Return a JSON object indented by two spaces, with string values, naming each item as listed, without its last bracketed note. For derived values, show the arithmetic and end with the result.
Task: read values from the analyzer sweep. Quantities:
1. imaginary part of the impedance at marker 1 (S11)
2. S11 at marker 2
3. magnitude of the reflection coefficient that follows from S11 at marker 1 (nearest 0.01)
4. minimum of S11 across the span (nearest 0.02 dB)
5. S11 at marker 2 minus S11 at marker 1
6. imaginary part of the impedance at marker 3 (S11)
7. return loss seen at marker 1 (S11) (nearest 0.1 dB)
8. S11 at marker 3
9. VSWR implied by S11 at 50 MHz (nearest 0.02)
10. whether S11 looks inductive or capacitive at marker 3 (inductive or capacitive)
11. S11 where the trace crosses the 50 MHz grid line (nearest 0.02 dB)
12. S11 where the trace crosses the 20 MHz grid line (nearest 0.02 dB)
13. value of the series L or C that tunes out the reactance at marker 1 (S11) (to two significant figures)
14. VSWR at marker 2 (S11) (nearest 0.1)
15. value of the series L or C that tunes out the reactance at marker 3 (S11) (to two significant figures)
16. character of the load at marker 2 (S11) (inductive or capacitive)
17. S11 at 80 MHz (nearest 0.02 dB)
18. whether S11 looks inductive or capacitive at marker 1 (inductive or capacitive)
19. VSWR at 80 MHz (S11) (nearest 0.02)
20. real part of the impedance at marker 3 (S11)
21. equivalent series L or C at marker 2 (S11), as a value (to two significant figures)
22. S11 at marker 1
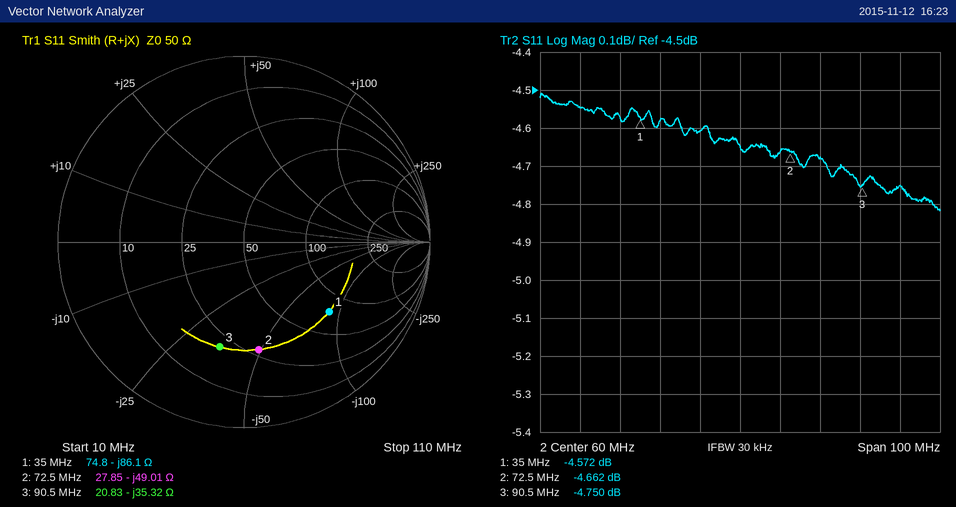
{
  "imaginary part of the impedance at marker 1": "-86.1 Ω",
  "S11 at marker 2": "-4.662 dB",
  "magnitude of the reflection coefficient that follows from S11 at marker 1": "10^(-4.572/20) ≈ 0.59",
  "minimum of S11 across the span": "-4.82 dB",
  "S11 at marker 2 minus S11 at marker 1": "-4.662 − (-4.572) = -0.090 dB",
  "imaginary part of the impedance at marker 3": "-35.32 Ω",
  "return loss seen at marker 1 (S11)": "4.6 dB",
  "S11 at marker 3": "-4.750 dB",
  "VSWR implied by S11 at 50 MHz": "|Γ| = 10^(-4.6/20) = 0.5888; VSWR = (1 + 0.5888)/(1 − 0.5888) ≈ 3.86",
  "whether S11 looks inductive or capacitive at marker 3": "capacitive",
  "S11 where the trace crosses the 50 MHz grid line": "-4.60 dB",
  "S11 where the trace crosses the 20 MHz grid line": "-4.54 dB",
  "value of the series L or C that tunes out the reactance at marker 1 (S11)": "L = 86.1 Ω/(2π × 35 MHz) ≈ 392 nH, so 390 nH to two significant figures",
  "VSWR at marker 2 (S11)": "3.8",
  "value of the series L or C that tunes out the reactance at marker 3 (S11)": "L = 35.32 Ω/(2π × 90.5 MHz) ≈ 62 nH",
  "character of the load at marker 2 (S11)": "capacitive",
  "S11 at 80 MHz": "-4.68 dB",
  "whether S11 looks inductive or capacitive at marker 1": "capacitive",
  "VSWR at 80 MHz (S11)": "|Γ| = 10^(-4.68/20) = 0.5834; VSWR = (1 + 0.5834)/(1 − 0.5834) ≈ 3.80",
  "real part of the impedance at marker 3": "20.83 Ω",
  "equivalent series L or C at marker 2 (S11), as a value": "C = 1/(2π × 72.5 MHz × 49.01 Ω) ≈ 45 pF",
  "S11 at marker 1": "-4.572 dB"
}
